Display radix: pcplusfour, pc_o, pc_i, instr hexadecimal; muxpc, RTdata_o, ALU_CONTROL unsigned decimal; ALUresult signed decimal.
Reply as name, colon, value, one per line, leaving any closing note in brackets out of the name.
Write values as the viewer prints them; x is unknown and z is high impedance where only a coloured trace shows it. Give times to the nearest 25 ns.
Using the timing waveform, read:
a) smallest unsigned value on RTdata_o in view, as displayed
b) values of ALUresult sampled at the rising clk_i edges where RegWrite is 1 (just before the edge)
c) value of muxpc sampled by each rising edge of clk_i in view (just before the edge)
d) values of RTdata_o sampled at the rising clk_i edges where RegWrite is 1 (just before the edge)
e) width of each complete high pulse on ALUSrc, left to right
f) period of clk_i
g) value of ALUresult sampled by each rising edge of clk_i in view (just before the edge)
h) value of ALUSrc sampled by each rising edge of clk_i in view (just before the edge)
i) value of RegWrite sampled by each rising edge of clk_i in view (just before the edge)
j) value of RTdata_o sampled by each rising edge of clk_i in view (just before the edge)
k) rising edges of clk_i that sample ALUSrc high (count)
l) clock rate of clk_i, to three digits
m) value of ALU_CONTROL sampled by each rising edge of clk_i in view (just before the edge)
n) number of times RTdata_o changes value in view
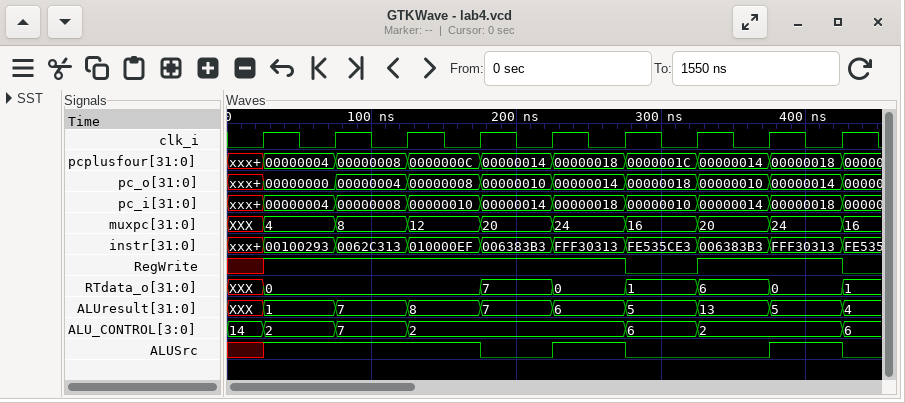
smallest unsigned value on RTdata_o in view, as displayed: 0
values of ALUresult sampled at the rising clk_i edges where RegWrite is 1: 1, 7, 8, 7, 6, 13, 5
value of muxpc sampled by each rising edge of clk_i in view: XXX, 4, 8, 12, 20, 24, 16, 20, 24
values of RTdata_o sampled at the rising clk_i edges where RegWrite is 1: 0, 0, 0, 7, 0, 6, 0
width of each complete high pulse on ALUSrc, left to right: 50 ns, 50 ns
period of clk_i: 50 ns
value of ALUresult sampled by each rising edge of clk_i in view: XXX, 1, 7, 8, 7, 6, 5, 13, 5
value of ALUSrc sampled by each rising edge of clk_i in view: x 1 1 1 0 1 0 0 1
value of RegWrite sampled by each rising edge of clk_i in view: x 1 1 1 1 1 0 1 1
value of RTdata_o sampled by each rising edge of clk_i in view: XXX, 0, 0, 0, 7, 0, 1, 6, 0
rising edges of clk_i that sample ALUSrc high: 5
clock rate of clk_i, to three digits: 20.0 MHz
value of ALU_CONTROL sampled by each rising edge of clk_i in view: 14, 2, 7, 2, 2, 2, 6, 2, 2
number of times RTdata_o changes value in view: 7
